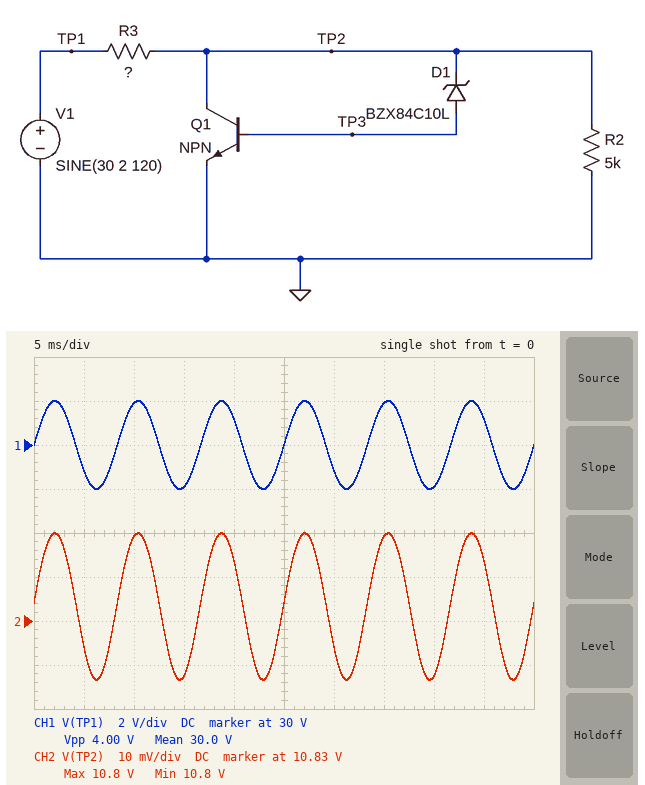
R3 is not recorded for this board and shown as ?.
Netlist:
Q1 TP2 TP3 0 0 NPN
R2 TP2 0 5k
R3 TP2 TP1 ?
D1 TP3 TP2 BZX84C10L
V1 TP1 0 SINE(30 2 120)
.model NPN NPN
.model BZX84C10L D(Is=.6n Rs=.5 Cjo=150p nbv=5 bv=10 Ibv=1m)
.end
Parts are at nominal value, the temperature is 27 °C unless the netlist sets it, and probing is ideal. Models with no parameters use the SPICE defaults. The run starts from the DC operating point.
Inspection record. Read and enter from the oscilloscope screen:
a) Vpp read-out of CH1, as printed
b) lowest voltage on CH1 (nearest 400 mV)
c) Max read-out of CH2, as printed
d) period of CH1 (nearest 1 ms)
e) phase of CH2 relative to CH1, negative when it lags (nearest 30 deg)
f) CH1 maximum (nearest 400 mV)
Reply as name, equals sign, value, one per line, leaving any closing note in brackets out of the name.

Vpp read-out of CH1, as printed = 4.00 V
lowest voltage on CH1 = 28.0 V
Max read-out of CH2, as printed = 10.8 V
period of CH1 = 8 ms
phase of CH2 relative to CH1, negative when it lags = 0 deg
CH1 maximum = 32.0 V
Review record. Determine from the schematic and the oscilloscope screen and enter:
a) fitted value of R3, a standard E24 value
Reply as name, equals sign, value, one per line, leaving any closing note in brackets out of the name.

fitted value of R3, a standard E24 value = 270 Ω
